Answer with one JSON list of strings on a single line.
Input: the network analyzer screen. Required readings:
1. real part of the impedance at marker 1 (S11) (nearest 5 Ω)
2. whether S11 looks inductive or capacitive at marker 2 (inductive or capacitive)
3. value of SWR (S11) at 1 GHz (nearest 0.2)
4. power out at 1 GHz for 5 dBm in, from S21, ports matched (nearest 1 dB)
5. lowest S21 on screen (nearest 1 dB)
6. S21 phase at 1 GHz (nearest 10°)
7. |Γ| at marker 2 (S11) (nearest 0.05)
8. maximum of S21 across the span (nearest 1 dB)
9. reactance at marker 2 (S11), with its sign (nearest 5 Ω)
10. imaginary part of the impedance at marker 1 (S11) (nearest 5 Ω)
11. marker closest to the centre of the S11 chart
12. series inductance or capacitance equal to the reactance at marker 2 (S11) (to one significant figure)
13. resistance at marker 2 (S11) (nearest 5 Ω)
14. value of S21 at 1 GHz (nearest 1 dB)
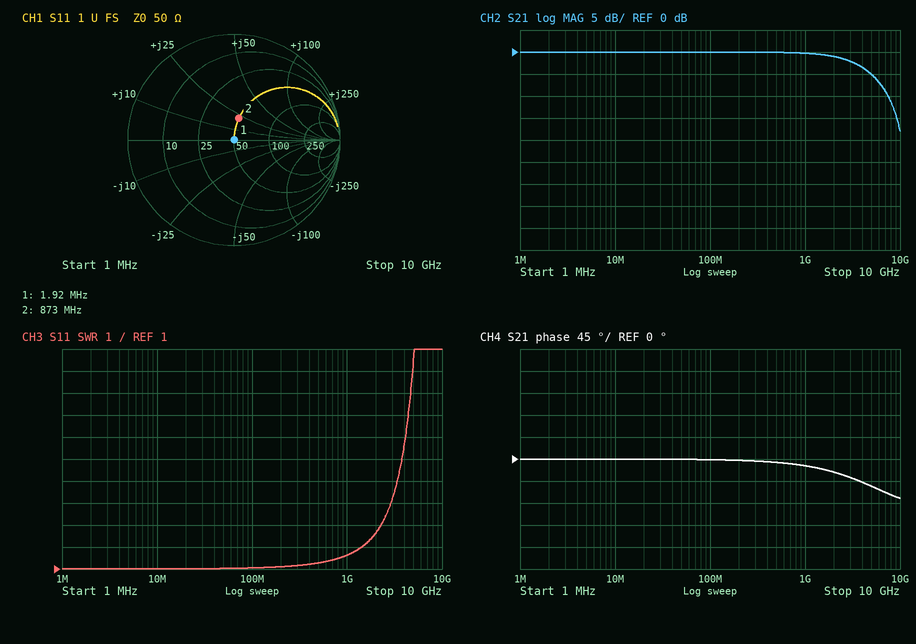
["50 Ω", "inductive", "1.6", "5 dBm", "-18 dB", "-10°", "0.20", "0 dB", "+20 Ω", "0 Ω", "marker 1", "4 nH", "50 Ω", "0 dB"]
